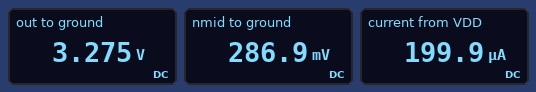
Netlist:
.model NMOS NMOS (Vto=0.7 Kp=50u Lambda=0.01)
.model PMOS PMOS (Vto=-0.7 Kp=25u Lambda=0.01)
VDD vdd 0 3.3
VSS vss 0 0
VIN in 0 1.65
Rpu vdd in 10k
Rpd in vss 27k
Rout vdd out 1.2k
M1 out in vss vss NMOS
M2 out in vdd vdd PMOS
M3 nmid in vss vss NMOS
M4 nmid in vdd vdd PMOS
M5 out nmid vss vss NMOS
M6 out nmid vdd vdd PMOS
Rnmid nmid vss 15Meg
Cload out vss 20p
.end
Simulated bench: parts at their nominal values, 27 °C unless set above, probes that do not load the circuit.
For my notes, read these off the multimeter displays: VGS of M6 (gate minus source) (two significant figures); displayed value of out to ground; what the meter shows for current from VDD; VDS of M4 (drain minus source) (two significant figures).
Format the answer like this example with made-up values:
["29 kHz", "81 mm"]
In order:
["-3.0 V", "3.275 V", "199.9 µA", "-3.0 V"]
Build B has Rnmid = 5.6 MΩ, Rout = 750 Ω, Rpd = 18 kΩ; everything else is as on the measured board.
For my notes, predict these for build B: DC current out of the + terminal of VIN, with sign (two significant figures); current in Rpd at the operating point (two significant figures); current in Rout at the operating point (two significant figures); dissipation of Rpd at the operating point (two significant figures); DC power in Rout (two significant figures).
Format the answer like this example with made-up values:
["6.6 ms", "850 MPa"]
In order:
["-73 µA", "92 µA", "22 µA", "150 µW", "360 nW"]
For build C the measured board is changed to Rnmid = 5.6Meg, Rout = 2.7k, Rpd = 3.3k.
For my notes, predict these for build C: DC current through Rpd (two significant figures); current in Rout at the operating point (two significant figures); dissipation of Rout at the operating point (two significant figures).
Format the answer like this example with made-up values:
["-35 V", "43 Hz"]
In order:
["500 µA", "19 µA", "990 nW"]
